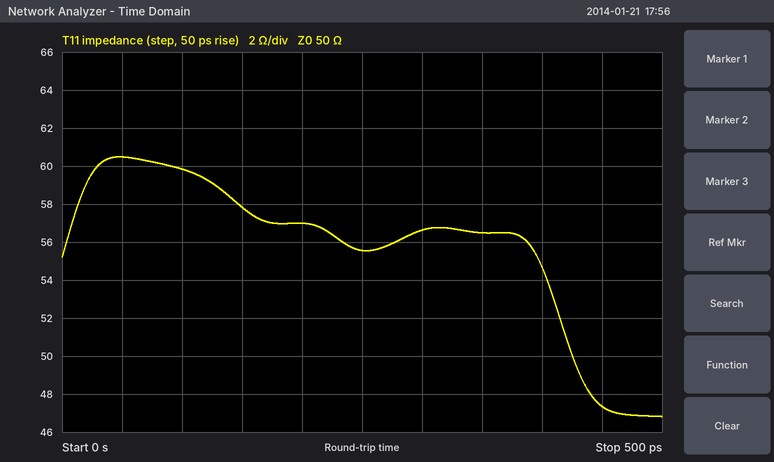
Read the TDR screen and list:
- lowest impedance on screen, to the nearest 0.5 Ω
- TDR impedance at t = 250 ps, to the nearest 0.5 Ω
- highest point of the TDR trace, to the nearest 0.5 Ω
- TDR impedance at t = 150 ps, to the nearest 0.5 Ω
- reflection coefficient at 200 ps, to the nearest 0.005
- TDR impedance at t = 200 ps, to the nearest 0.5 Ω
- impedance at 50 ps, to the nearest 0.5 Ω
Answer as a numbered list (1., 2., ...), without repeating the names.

1. 47.0 Ω
2. 55.5 Ω
3. 60.5 Ω
4. 58.0 Ω
5. +0.065
6. 57.0 Ω
7. 60.5 Ω
